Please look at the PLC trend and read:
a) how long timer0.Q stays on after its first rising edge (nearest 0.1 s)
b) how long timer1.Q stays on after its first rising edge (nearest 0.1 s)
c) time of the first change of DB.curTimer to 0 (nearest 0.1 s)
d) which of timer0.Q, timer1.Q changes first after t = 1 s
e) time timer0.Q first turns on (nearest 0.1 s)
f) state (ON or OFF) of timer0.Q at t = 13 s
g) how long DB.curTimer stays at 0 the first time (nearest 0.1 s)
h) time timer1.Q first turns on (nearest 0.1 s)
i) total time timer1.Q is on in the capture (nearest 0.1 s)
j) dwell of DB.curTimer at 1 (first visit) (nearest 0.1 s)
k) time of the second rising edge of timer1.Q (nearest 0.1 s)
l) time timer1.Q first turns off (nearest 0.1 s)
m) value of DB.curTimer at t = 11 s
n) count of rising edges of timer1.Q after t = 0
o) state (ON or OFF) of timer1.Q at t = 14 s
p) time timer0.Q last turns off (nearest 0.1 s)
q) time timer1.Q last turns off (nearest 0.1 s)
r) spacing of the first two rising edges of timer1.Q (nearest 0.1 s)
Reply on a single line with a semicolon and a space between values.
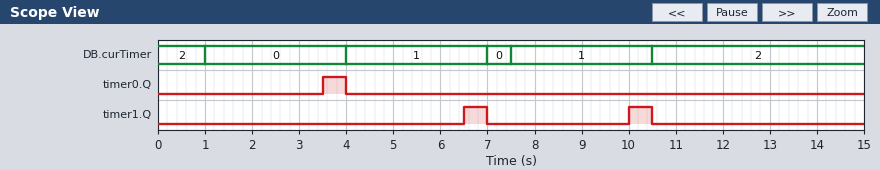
0.5 s; 0.5 s; 1.0 s; timer0.Q; 3.5 s; OFF; 3.0 s; 6.5 s; 1.0 s; 3.0 s; 10.0 s; 7.0 s; 2; 2; OFF; 4.0 s; 10.5 s; 3.5 s
